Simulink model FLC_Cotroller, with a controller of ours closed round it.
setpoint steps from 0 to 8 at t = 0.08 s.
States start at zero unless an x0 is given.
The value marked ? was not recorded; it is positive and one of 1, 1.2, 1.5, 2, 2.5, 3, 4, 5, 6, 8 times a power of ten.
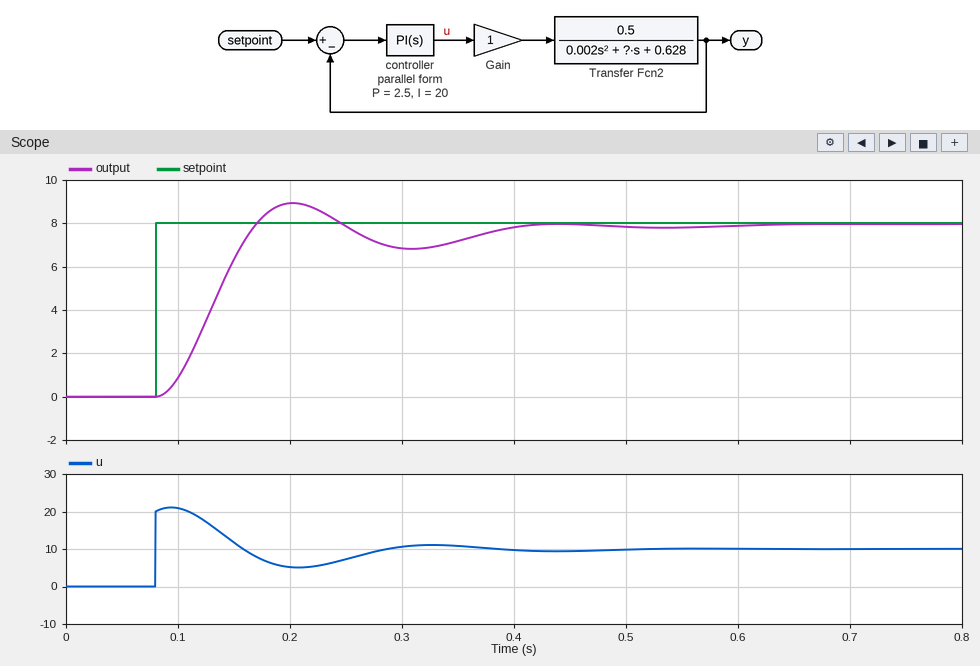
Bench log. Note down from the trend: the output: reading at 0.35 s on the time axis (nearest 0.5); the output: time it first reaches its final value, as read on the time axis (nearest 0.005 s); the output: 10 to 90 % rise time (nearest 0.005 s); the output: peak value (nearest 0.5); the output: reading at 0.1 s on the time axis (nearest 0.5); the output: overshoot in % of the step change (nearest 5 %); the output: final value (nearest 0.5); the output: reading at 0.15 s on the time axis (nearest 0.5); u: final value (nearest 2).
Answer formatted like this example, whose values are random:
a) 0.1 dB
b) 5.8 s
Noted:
a) 7.0
b) 0.170 s
c) 0.060 s
d) 9.0
e) 1.0
f) 10 %
g) 8.0
h) 6.5
i) 10
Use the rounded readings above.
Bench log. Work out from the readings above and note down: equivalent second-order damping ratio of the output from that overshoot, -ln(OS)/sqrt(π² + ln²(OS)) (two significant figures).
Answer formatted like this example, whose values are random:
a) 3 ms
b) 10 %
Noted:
a) 0.59
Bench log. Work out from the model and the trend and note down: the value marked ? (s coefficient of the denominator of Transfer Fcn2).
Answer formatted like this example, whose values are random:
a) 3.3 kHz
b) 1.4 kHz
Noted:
a) 0.05
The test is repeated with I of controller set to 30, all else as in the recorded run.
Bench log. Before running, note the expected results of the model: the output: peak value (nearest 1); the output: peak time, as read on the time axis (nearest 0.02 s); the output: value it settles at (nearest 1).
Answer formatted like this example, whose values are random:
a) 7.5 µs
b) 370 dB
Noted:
a) 10
b) 0.20 s
c) 8
